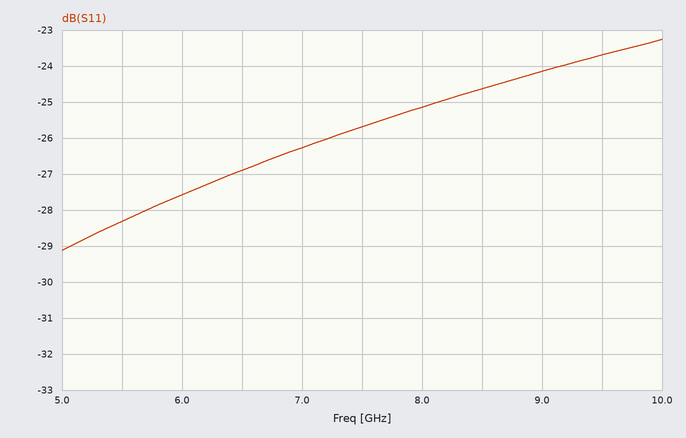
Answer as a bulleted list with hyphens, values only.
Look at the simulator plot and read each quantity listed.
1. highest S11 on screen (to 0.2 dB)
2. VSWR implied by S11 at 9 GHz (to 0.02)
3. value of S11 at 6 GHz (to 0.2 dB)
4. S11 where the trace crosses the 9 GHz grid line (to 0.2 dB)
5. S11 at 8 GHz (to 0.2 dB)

- -23.2 dB
- 1.14
- -27.6 dB
- -24.2 dB
- -25.2 dB
